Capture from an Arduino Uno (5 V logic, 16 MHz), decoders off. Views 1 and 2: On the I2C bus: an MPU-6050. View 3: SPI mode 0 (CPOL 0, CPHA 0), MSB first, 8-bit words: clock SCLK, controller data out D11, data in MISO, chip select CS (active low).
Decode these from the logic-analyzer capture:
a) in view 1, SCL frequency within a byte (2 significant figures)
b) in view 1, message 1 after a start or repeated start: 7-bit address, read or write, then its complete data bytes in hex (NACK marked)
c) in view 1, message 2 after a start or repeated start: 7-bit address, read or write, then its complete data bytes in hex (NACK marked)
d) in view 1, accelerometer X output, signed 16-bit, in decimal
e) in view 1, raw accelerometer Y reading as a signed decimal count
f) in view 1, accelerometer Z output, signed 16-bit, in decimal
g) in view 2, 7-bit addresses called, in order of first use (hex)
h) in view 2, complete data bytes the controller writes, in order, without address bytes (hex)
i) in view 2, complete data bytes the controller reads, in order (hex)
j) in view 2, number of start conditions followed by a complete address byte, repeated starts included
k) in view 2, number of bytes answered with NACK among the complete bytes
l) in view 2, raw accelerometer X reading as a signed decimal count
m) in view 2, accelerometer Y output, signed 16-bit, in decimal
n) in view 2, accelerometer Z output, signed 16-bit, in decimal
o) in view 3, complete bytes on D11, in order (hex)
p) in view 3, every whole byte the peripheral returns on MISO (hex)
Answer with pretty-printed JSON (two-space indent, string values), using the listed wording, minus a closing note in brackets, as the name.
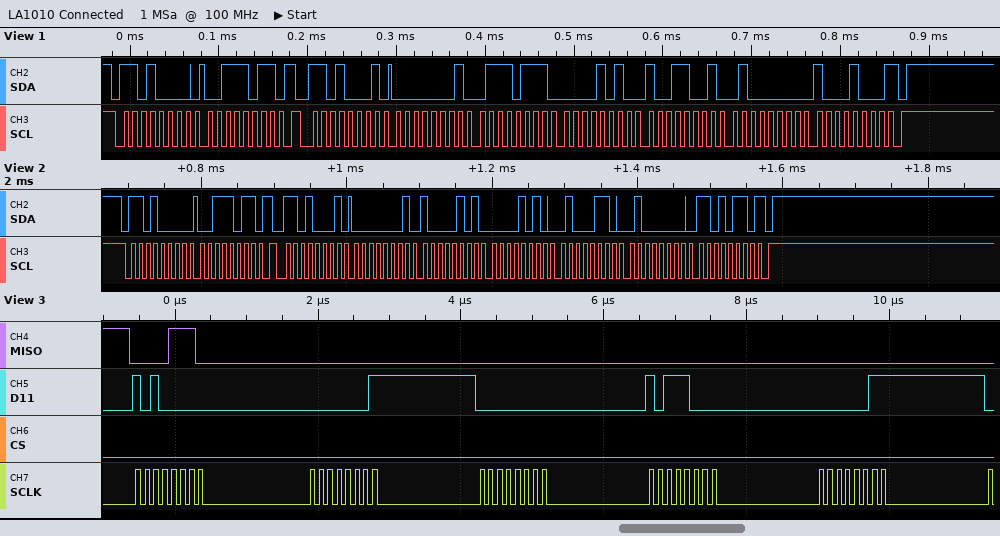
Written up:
{
  "in view 1, SCL frequency within a byte": "100 kHz",
  "in view 1, message 1 after a start or repeated start: 7-bit address, read or write, then its complete data bytes in hex": "0x68 write: 3B",
  "in view 1, message 2 after a start or repeated start: 7-bit address, read or write, then its complete data bytes in hex": "0x68 read: 01 77 0A 99 40 88 NACK",
  "in view 1, accelerometer X output, signed 16-bit, in decimal": "375",
  "in view 1, raw accelerometer Y reading as a signed decimal count": "2713",
  "in view 1, accelerometer Z output, signed 16-bit, in decimal": "16520",
  "in view 2, 7-bit addresses called, in order of first use": "0x68",
  "in view 2, complete data bytes the controller writes, in order, without address bytes": "3B",
  "in view 2, complete data bytes the controller reads, in order": "01 85 0A 46 40 D6",
  "in view 2, number of start conditions followed by a complete address byte, repeated starts included": "2",
  "in view 2, number of bytes answered with NACK among the complete bytes": "1",
  "in view 2, raw accelerometer X reading as a signed decimal count": "389",
  "in view 2, accelerometer Y output, signed 16-bit, in decimal": "2630",
  "in view 2, accelerometer Z output, signed 16-bit, in decimal": "16598",
  "in view 3, complete bytes on D11, in order": "A0 01 00 B8 03",
  "in view 3, every whole byte the peripheral returns on MISO": "0E 00 00 00 00"
}
